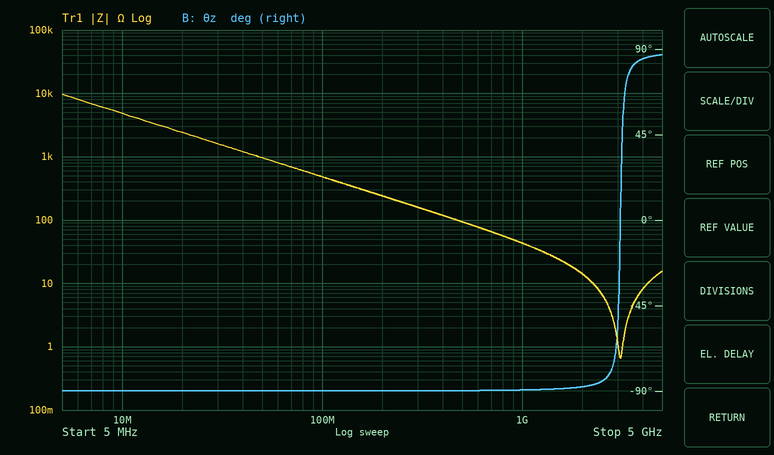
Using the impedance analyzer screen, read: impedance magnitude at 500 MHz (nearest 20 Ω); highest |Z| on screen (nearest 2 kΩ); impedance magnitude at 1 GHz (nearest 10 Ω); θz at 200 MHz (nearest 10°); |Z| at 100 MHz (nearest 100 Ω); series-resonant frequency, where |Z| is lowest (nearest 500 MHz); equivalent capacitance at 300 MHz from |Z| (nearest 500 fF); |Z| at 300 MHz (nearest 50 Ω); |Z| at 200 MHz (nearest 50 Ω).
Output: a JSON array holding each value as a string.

["100 Ω", "10 kΩ", "40 Ω", "-90°", "500 Ω", "3.0 GHz", "3.5 pF", "150 Ω", "250 Ω"]
